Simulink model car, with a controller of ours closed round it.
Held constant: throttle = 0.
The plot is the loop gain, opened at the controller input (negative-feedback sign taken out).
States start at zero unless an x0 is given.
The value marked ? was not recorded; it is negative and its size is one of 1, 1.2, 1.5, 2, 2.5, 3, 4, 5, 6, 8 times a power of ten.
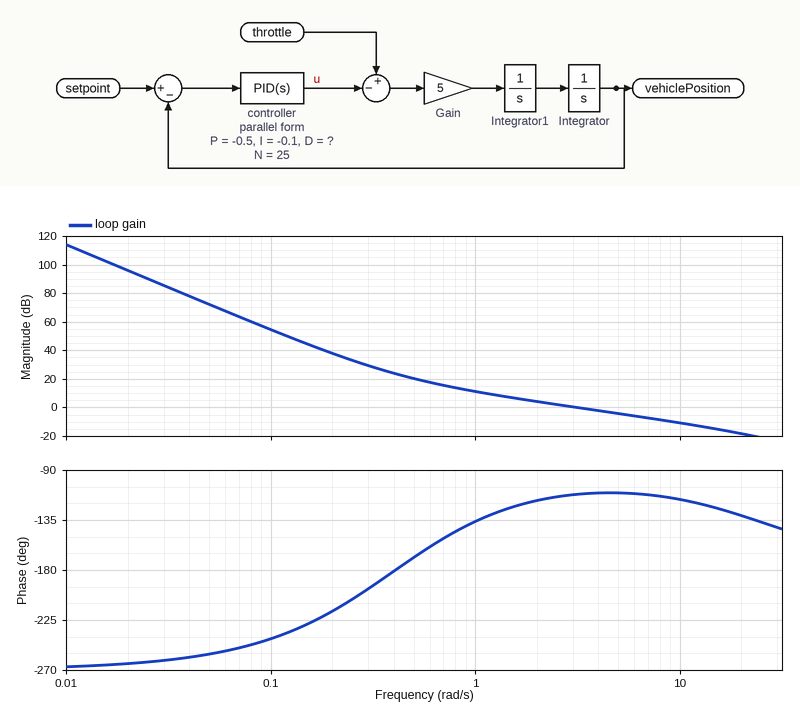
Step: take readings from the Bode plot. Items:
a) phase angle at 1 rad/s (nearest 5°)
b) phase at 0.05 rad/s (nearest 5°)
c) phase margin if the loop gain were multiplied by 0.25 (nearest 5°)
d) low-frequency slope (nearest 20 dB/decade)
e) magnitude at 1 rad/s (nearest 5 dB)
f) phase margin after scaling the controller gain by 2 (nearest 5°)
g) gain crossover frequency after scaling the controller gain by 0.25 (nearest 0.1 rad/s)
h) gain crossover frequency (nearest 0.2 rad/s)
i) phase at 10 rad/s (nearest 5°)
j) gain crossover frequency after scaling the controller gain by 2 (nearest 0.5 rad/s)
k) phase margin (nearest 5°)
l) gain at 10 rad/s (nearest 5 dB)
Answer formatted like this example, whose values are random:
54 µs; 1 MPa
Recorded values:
-135°; -255°; 40°; -60 dB/decade; 10 dB; 70°; 0.9 rad/s; 3.2 rad/s; -115°; 6.0 rad/s; 70°; -10 dB
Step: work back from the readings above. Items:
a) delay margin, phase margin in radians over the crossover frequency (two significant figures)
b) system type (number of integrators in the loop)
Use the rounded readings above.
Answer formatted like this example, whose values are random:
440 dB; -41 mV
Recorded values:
0.38 s; 3
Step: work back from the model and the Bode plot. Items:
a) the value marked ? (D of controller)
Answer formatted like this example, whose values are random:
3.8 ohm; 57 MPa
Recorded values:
-0.6
